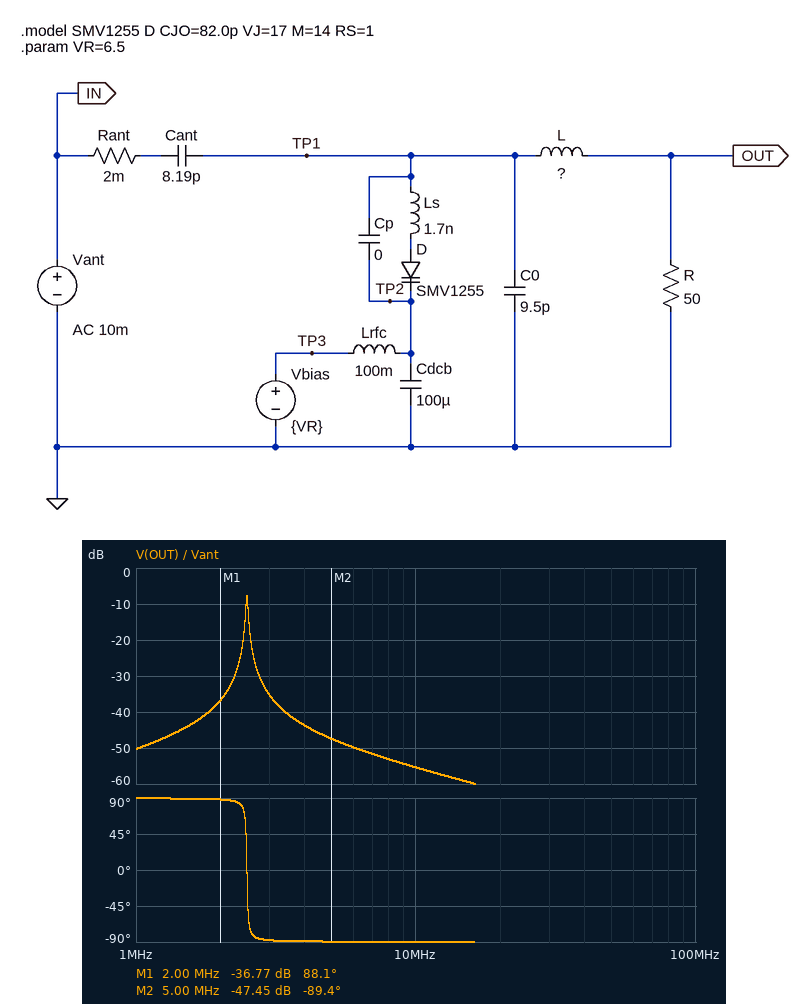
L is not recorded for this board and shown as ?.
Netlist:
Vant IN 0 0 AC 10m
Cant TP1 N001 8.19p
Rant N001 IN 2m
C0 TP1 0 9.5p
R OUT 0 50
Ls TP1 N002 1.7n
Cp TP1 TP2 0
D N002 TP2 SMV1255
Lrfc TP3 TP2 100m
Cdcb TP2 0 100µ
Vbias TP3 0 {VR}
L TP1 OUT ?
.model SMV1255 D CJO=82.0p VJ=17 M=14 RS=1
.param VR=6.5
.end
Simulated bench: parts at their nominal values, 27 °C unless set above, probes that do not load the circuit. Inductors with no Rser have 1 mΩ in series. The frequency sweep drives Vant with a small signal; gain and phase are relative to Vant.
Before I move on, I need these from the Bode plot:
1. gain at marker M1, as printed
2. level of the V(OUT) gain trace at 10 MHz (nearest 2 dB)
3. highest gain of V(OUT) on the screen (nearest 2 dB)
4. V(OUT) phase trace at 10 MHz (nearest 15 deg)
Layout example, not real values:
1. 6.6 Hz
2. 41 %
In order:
1. -36.77 dB
2. -56 dB
3. -8 dB
4. -90 deg
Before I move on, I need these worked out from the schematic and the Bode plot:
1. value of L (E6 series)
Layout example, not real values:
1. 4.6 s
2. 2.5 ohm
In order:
1. 220 µH
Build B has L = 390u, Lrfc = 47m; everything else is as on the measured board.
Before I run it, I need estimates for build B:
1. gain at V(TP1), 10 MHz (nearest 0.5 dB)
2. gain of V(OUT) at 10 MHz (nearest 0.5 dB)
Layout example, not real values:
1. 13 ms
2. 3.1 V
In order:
1. -7.0 dB
2. -60.5 dB
